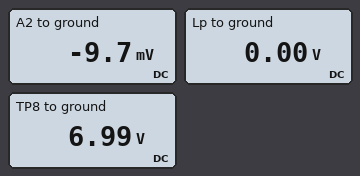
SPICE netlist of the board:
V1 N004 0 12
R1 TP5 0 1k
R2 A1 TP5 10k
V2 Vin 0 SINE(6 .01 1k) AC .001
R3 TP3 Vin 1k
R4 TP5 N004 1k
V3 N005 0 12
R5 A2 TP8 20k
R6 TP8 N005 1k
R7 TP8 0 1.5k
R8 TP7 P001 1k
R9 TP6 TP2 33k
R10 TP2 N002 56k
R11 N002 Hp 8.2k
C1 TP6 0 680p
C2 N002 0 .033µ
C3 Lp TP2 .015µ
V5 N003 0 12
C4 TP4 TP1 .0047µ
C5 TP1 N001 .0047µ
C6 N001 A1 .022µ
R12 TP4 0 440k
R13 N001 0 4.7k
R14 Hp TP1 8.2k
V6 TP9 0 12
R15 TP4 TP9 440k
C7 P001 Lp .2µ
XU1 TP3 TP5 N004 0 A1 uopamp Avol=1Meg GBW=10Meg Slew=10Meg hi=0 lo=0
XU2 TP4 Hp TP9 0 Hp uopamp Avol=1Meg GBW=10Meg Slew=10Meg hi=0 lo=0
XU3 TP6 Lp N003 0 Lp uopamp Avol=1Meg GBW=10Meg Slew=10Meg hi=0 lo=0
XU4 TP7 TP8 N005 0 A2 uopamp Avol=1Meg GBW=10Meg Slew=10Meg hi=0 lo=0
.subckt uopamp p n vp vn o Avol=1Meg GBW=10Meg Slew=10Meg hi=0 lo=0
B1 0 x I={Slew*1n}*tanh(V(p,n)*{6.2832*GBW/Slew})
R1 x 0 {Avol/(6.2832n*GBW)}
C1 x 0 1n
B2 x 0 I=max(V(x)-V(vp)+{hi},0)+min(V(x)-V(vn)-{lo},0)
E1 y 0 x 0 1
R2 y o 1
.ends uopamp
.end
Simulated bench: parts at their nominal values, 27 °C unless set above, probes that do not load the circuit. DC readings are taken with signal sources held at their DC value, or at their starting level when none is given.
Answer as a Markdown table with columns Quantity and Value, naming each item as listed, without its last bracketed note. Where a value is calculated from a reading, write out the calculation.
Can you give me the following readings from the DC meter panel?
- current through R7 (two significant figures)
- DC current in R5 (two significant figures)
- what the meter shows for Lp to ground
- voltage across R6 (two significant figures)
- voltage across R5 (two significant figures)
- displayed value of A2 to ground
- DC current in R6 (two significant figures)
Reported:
| Quantity | Value |
|---|---|
| current through R7 | (6.99 V) / 1.5 kΩ = 4.7 mA |
| DC current in R5 | (6.99 V - (-9.7 mV)) / 20 kΩ = 350 µA |
| what the meter shows for Lp to ground | 0.00 V |
| voltage across R6 | 12 V - 6.99 V = 5.0 V |
| voltage across R5 | 6.99 V - (-9.7 mV) = 7.0 V |
| displayed value of A2 to ground | -9.7 mV |
| DC current in R6 | (12 V - 6.99 V) / 1 kΩ = 5.0 mA |
